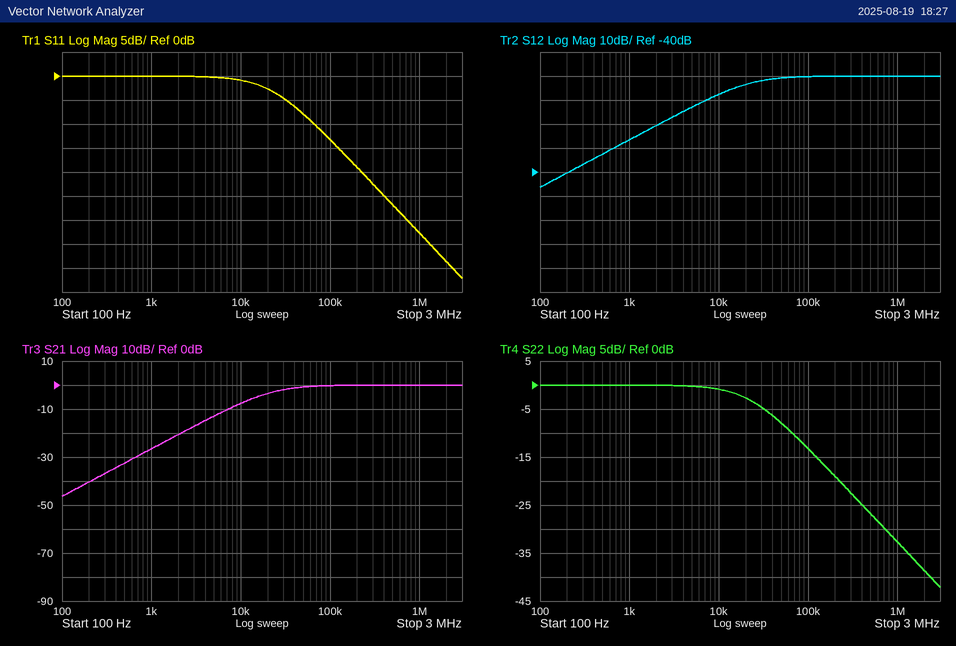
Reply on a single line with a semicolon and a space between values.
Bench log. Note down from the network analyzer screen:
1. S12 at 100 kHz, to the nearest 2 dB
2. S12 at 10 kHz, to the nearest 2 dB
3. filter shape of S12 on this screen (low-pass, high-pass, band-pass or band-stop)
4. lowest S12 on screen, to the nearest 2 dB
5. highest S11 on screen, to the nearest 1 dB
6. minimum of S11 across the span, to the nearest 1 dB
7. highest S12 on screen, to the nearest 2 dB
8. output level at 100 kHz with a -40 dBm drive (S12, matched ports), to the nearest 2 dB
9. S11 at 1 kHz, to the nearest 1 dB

0 dB; -8 dB; high-pass; -46 dB; 0 dB; -42 dB; 0 dB; -40 dBm; 0 dB
